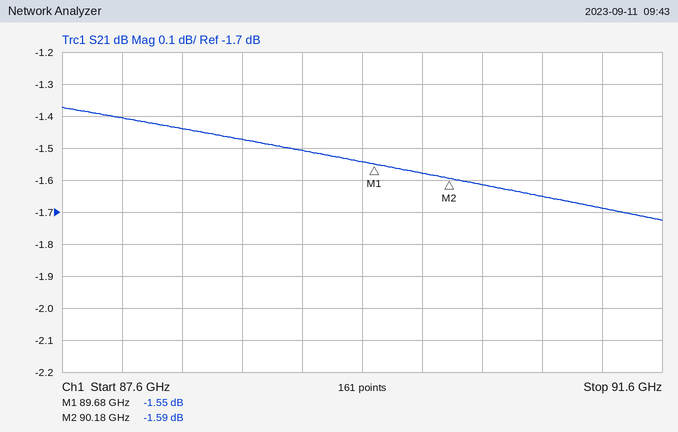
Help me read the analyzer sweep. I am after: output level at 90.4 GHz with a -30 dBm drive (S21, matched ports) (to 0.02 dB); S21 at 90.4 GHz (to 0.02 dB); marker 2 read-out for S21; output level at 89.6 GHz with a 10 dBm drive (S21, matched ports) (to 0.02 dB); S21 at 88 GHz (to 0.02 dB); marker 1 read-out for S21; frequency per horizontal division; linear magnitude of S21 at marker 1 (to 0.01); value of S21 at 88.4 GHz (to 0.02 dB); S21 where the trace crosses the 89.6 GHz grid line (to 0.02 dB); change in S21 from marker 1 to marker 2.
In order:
-31.62 dBm
-1.62 dB
-1.59 dB
8.46 dBm
-1.40 dB
-1.55 dB
400 MHz
0.84
-1.44 dB
-1.54 dB
-0.04 dB
